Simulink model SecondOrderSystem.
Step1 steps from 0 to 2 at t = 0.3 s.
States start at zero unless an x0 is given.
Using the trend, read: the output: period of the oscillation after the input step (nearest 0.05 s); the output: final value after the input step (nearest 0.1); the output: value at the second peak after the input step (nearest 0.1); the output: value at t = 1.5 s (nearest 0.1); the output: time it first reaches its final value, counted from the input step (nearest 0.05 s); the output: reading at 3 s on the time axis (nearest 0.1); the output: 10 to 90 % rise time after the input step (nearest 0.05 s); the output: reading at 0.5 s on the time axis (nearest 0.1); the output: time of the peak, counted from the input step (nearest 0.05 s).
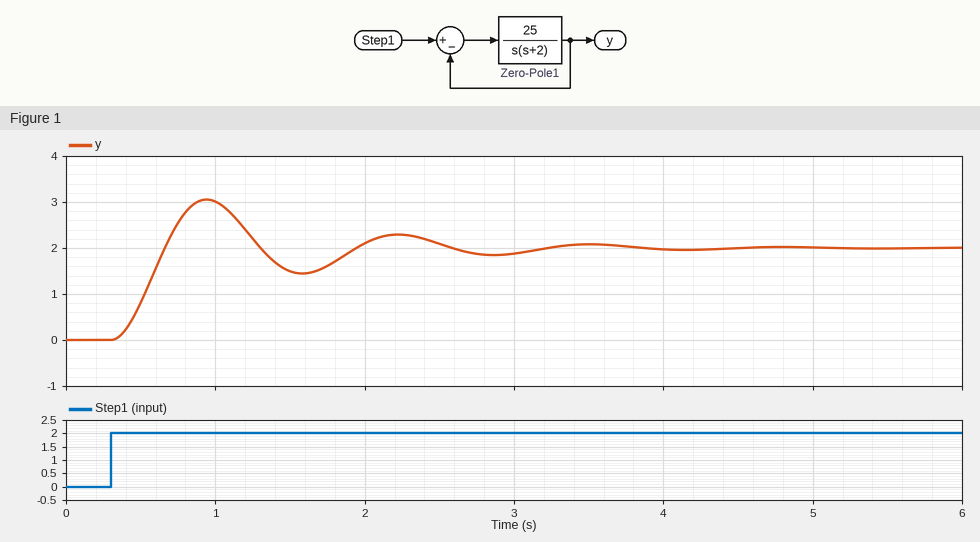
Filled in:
1.30 s
2.0
2.3
1.5
0.35 s
1.9
0.25 s
0.8
0.65 s
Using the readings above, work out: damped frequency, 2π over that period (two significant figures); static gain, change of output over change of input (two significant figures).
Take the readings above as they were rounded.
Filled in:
4.8 rad/s
1.0
